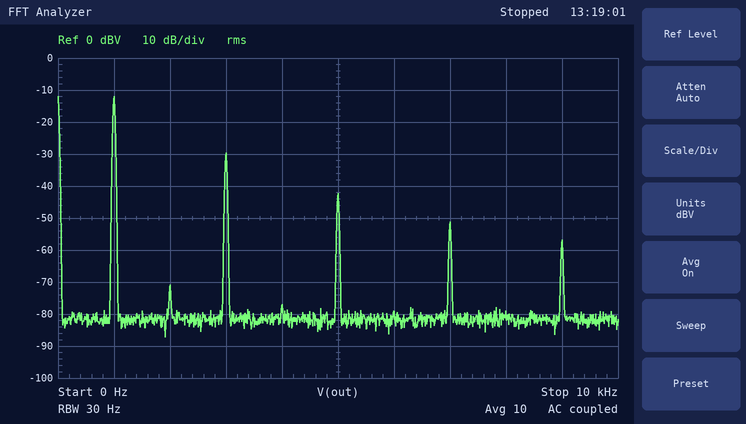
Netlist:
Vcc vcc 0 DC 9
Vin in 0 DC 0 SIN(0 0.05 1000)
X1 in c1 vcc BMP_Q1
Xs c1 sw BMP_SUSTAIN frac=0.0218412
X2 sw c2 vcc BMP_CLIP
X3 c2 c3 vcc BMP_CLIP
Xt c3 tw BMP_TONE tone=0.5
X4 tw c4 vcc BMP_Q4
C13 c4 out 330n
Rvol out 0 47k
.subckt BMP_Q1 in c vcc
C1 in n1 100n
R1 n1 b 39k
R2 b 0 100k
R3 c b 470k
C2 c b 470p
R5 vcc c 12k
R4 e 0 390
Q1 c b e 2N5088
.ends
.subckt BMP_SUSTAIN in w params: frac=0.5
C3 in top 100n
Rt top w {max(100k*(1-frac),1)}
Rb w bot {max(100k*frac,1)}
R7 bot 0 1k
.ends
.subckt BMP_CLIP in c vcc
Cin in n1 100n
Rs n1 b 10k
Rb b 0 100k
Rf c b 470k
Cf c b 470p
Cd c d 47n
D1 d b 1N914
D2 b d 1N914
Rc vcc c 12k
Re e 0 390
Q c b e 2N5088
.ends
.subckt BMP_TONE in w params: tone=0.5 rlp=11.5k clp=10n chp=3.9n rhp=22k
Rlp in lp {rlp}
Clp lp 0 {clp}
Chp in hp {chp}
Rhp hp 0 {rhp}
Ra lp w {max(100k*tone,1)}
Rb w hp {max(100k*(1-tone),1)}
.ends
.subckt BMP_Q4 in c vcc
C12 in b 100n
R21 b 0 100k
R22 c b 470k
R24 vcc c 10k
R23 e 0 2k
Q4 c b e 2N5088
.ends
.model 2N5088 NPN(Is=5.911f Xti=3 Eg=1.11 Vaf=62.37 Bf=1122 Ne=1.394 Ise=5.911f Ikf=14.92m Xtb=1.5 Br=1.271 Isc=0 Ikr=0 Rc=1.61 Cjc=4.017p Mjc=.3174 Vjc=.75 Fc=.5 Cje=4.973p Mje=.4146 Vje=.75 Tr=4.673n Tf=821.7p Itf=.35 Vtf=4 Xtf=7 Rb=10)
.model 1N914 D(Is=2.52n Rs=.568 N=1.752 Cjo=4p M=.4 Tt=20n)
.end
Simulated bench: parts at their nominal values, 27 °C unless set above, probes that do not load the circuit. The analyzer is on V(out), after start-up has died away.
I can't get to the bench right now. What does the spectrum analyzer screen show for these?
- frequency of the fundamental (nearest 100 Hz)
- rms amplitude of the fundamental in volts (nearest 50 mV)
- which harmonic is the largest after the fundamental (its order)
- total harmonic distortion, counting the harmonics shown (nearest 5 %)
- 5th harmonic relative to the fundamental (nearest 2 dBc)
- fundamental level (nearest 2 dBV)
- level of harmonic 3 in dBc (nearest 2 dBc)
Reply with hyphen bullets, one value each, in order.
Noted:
- 1.0 kHz
- 250 mV
- 3
- 15 %
- -30 dBc
- -12 dBV
- -18 dBc
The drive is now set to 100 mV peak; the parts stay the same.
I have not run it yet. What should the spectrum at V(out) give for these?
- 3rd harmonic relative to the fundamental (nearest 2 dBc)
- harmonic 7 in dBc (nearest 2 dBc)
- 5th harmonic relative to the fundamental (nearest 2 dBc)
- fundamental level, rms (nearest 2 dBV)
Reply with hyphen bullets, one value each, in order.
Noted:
- -14 dBc
- -30 dBc
- -22 dBc
- -10 dBV
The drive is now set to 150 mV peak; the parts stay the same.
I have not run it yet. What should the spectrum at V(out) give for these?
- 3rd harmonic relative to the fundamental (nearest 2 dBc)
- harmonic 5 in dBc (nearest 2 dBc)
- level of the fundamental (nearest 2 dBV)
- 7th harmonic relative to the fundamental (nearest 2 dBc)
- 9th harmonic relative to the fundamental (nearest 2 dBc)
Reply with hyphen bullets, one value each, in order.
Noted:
- -14 dBc
- -20 dBc
- -10 dBV
- -26 dBc
- -32 dBc
